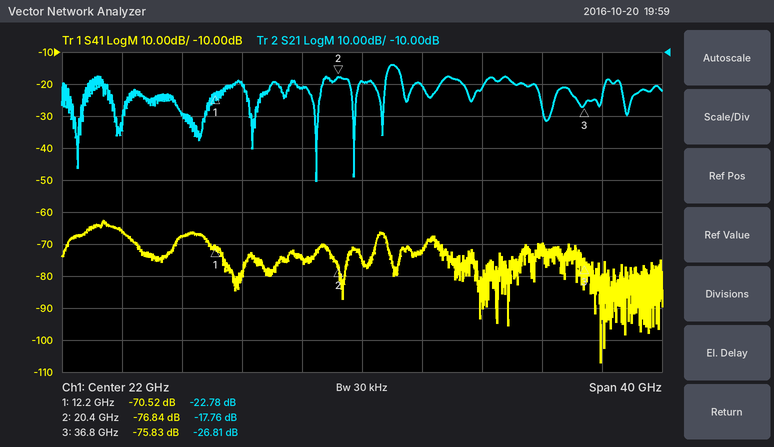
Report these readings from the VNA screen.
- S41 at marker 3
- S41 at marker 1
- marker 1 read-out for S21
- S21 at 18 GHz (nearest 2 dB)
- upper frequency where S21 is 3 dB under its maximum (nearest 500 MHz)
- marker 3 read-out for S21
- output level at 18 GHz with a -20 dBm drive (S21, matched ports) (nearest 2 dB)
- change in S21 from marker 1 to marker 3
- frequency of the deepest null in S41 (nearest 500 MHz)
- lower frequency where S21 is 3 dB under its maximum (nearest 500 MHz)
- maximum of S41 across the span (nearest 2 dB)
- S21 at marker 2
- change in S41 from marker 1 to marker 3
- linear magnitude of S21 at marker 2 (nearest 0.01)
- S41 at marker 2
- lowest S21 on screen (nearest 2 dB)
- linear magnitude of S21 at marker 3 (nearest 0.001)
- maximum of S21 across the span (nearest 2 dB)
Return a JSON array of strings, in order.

["-75.83 dB", "-70.52 dB", "-22.78 dB", "-22 dB", "24.5 GHz", "-26.81 dB", "-42 dBm", "-4.03 dB", "38.0 GHz", "23.5 GHz", "-62 dB", "-17.76 dB", "-5.31 dB", "0.13", "-76.84 dB", "-50 dB", "0.046", "-14 dB"]
